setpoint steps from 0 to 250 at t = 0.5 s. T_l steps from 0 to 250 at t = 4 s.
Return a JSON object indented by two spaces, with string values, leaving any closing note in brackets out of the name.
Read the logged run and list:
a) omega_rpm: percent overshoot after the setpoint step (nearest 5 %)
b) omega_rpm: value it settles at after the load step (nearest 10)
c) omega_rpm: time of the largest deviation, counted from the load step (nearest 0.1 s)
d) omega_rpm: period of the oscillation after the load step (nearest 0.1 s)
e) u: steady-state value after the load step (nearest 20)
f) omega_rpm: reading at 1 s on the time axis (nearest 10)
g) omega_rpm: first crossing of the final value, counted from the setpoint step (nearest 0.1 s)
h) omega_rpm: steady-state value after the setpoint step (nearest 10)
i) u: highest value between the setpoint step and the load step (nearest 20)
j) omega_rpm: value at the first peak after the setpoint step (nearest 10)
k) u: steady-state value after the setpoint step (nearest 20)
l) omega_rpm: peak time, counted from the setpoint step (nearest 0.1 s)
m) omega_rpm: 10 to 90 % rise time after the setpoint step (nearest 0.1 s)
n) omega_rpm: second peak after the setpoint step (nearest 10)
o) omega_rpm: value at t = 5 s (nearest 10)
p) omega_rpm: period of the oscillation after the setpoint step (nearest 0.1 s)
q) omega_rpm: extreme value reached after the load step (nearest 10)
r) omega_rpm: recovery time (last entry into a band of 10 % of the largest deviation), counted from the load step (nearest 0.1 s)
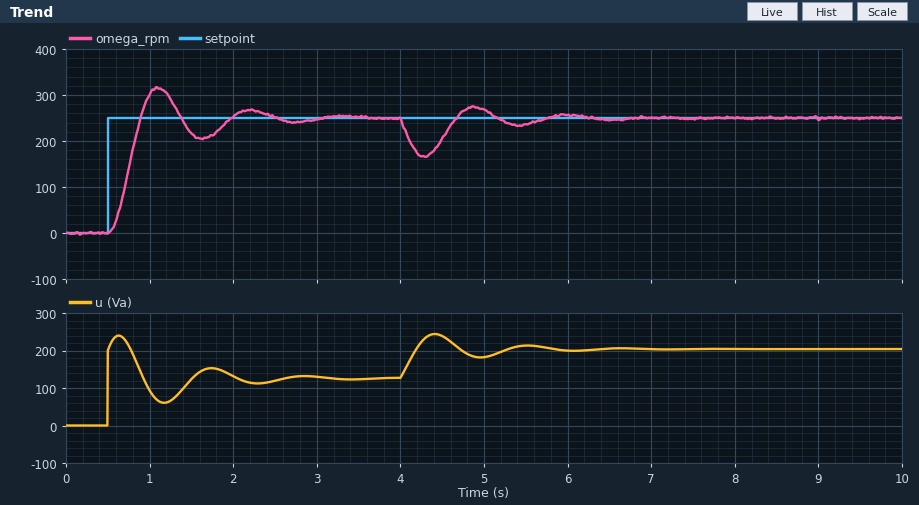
{
  "omega_rpm: percent overshoot after the setpoint step": "25 %",
  "omega_rpm: value it settles at after the load step": "250",
  "omega_rpm: time of the largest deviation, counted from the load step": "0.3 s",
  "omega_rpm: period of the oscillation after the load step": "1.1 s",
  "u: steady-state value after the load step": "200",
  "omega_rpm: reading at 1 s on the time axis": "300",
  "omega_rpm: first crossing of the final value, counted from the setpoint step": "0.4 s",
  "omega_rpm: steady-state value after the setpoint step": "250",
  "u: highest value between the setpoint step and the load step": "240",
  "omega_rpm: value at the first peak after the setpoint step": "320",
  "u: steady-state value after the setpoint step": "120",
  "omega_rpm: peak time, counted from the setpoint step": "0.6 s",
  "omega_rpm: 10 to 90 % rise time after the setpoint step": "0.3 s",
  "omega_rpm: second peak after the setpoint step": "270",
  "omega_rpm: value at t = 5 s": "270",
  "omega_rpm: period of the oscillation after the setpoint step": "1.1 s",
  "omega_rpm: extreme value reached after the load step": "170",
  "omega_rpm: recovery time (last entry into a band of 10 % of the largest deviation), counted from the load step": "1.6 s"
}
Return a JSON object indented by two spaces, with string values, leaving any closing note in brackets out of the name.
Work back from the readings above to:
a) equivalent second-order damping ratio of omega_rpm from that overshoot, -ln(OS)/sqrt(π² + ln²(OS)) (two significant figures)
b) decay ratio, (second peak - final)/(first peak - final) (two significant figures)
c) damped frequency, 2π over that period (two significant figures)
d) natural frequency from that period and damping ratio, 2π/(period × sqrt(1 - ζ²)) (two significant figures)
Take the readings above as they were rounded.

{
  "equivalent second-order damping ratio of omega_rpm from that overshoot, -ln(OS)/sqrt(π² + ln²(OS))": "0.40",
  "decay ratio, (second peak - final)/(first peak - final)": "0.29",
  "damped frequency, 2π over that period": "5.7 rad/s",
  "natural frequency from that period and damping ratio, 2π/(period × sqrt(1 - ζ²))": "6.2 rad/s"
}
